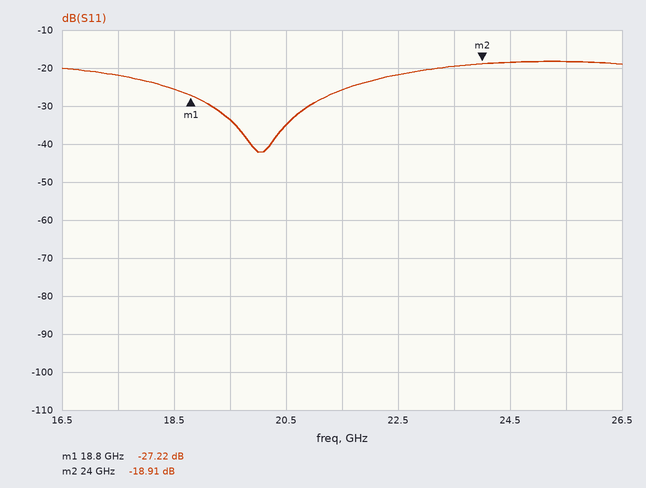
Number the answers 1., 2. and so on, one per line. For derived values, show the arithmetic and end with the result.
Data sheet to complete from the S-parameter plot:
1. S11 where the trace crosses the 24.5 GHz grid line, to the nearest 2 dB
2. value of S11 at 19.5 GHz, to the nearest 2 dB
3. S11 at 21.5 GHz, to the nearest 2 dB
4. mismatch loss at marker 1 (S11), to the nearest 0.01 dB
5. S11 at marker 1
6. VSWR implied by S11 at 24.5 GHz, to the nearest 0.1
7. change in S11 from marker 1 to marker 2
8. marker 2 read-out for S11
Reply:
1. -18 dB
2. -34 dB
3. -26 dB
4. −10 log10(1 − 10^(-27.22/10)) ≈ 0.01 dB
5. -27.22 dB
6. |Γ| = 10^(-18/20) = 0.1259; VSWR = (1 + 0.1259)/(1 − 0.1259) ≈ 1.3
7. -18.91 − (-27.22) = 8.31 dB
8. -18.91 dB
